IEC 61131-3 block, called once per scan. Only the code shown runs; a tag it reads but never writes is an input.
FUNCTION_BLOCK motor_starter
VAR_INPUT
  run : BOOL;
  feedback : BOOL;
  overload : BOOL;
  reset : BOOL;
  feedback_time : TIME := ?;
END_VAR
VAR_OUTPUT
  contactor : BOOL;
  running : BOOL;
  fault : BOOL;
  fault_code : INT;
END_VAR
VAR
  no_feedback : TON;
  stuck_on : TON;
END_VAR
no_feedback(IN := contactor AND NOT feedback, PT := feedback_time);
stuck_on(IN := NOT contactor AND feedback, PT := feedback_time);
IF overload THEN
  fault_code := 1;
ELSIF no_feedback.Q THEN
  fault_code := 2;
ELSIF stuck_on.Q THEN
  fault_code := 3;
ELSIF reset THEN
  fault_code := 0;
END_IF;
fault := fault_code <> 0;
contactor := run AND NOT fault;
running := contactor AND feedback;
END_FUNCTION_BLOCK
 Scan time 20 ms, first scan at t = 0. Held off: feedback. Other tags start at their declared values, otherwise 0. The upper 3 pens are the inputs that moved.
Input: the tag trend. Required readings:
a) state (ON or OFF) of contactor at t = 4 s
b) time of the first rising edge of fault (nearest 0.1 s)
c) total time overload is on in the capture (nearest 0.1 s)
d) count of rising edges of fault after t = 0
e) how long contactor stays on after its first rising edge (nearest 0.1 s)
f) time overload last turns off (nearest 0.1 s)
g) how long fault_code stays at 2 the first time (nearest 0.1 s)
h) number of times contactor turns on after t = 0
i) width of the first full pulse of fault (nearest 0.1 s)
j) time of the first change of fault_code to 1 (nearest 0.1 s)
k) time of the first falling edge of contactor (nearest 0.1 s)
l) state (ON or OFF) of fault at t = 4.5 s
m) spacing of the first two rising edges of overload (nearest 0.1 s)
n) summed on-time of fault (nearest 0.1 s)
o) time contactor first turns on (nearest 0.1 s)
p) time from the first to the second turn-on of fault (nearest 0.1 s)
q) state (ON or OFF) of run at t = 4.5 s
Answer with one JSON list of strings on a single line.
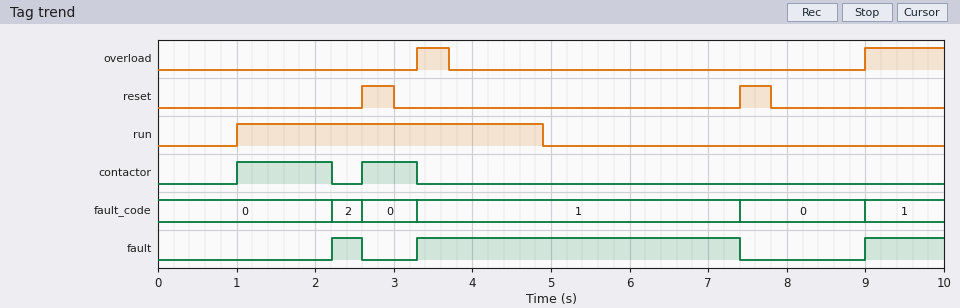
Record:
["OFF", "2.2 s", "1.4 s", "3", "1.2 s", "3.7 s", "0.4 s", "2", "0.4 s", "3.3 s", "2.2 s", "ON", "5.7 s", "5.5 s", "1.0 s", "1.1 s", "ON"]
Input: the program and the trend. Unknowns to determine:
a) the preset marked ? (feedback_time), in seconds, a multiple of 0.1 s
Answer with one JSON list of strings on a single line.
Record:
["1.2 s"]
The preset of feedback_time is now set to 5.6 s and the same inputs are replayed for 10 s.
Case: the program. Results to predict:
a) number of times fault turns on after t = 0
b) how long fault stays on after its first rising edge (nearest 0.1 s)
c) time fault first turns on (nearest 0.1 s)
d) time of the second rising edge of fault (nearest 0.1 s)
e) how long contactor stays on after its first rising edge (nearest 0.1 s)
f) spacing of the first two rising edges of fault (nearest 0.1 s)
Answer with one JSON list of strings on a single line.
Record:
["2", "4.1 s", "3.3 s", "9.0 s", "2.3 s", "5.7 s"]
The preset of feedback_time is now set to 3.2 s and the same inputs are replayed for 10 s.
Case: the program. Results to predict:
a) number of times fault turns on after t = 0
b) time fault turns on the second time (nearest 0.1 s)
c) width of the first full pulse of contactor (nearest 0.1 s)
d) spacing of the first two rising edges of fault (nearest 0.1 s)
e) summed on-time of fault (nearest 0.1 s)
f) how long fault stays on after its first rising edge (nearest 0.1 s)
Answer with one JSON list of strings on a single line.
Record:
["2", "9.0 s", "2.3 s", "5.7 s", "5.1 s", "4.1 s"]
